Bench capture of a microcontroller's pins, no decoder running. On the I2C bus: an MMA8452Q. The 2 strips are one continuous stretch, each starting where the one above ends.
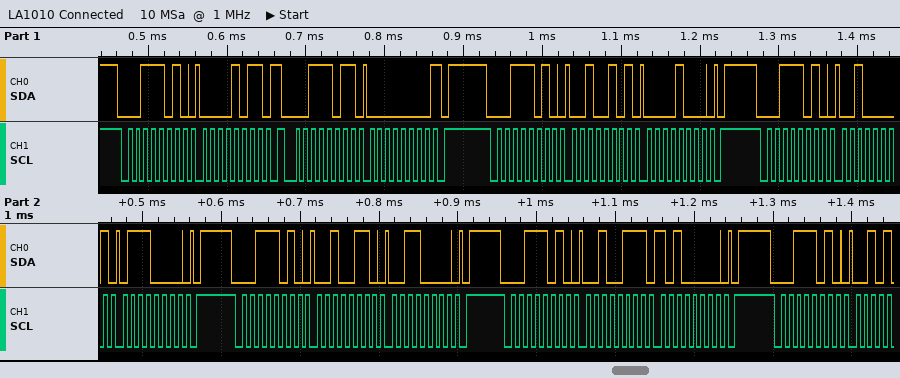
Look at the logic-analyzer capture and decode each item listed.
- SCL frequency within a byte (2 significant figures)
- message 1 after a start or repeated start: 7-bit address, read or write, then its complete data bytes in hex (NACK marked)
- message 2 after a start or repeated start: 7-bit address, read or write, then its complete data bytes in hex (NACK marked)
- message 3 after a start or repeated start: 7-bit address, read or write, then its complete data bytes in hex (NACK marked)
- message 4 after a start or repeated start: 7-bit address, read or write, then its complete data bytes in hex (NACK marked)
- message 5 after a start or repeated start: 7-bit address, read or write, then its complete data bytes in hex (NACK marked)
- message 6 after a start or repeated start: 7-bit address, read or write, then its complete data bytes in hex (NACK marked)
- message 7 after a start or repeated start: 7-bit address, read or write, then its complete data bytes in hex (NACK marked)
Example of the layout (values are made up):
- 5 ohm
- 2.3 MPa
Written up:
- 100 kHz
- 0x1D write: 0B
- 0x1D read: 00 NACK
- 0x1D write: 25 08
- 0x1D write: 21 70
- 0x1D write: 26 30
- 0x1D write: 27 A0
- 0x1D write
